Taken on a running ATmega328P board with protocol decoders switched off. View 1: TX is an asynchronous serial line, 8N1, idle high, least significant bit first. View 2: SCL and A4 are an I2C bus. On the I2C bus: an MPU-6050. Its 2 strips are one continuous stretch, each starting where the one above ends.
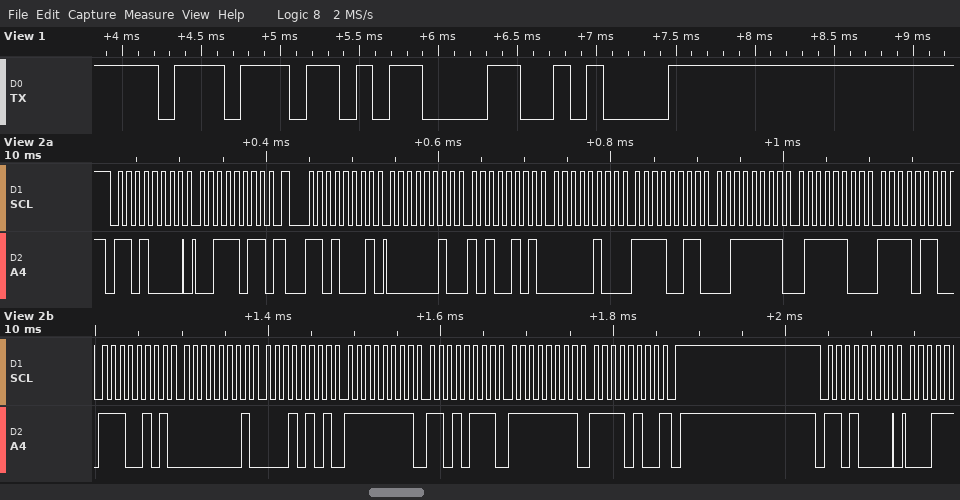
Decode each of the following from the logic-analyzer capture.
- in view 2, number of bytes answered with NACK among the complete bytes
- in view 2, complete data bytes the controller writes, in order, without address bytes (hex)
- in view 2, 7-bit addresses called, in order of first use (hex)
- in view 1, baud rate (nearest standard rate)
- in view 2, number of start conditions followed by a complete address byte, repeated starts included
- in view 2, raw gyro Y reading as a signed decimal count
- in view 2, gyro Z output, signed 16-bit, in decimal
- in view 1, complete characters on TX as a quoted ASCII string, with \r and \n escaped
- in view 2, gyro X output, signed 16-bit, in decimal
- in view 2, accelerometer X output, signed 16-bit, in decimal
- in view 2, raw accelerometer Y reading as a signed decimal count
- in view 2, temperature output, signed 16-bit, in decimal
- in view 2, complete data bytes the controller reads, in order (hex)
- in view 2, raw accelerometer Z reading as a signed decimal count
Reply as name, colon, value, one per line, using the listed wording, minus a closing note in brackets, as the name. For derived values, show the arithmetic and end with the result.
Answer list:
in view 2, number of bytes answered with NACK among the complete bytes: 1
in view 2, complete data bytes the controller writes, in order, without address bytes: 3B
in view 2, 7-bit addresses called, in order of first use: 0x68
in view 1, baud rate: 9600 baud
in view 2, number of start conditions followed by a complete address byte, repeated starts included: 3
in view 2, raw gyro Y reading as a signed decimal count: 0xFFD7 = -41
in view 2, gyro Z output, signed 16-bit, in decimal: 0xFFF4 = -12
in view 1, complete characters on TX as a quoted ASCII string, with \r and \n escaped: "w\r\n"
in view 2, gyro X output, signed 16-bit, in decimal: 0x0115 = 277
in view 2, accelerometer X output, signed 16-bit, in decimal: 0x02A5 = 677
in view 2, raw accelerometer Y reading as a signed decimal count: 0x04F3 = 1267
in view 2, temperature output, signed 16-bit, in decimal: 0xF6E5 = -2331
in view 2, complete data bytes the controller reads, in order: 02 A5 04 F3 3F 7C F6 E5 01 15 FF D7 FF F4
in view 2, raw accelerometer Z reading as a signed decimal count: 0x3F7C = 16252
